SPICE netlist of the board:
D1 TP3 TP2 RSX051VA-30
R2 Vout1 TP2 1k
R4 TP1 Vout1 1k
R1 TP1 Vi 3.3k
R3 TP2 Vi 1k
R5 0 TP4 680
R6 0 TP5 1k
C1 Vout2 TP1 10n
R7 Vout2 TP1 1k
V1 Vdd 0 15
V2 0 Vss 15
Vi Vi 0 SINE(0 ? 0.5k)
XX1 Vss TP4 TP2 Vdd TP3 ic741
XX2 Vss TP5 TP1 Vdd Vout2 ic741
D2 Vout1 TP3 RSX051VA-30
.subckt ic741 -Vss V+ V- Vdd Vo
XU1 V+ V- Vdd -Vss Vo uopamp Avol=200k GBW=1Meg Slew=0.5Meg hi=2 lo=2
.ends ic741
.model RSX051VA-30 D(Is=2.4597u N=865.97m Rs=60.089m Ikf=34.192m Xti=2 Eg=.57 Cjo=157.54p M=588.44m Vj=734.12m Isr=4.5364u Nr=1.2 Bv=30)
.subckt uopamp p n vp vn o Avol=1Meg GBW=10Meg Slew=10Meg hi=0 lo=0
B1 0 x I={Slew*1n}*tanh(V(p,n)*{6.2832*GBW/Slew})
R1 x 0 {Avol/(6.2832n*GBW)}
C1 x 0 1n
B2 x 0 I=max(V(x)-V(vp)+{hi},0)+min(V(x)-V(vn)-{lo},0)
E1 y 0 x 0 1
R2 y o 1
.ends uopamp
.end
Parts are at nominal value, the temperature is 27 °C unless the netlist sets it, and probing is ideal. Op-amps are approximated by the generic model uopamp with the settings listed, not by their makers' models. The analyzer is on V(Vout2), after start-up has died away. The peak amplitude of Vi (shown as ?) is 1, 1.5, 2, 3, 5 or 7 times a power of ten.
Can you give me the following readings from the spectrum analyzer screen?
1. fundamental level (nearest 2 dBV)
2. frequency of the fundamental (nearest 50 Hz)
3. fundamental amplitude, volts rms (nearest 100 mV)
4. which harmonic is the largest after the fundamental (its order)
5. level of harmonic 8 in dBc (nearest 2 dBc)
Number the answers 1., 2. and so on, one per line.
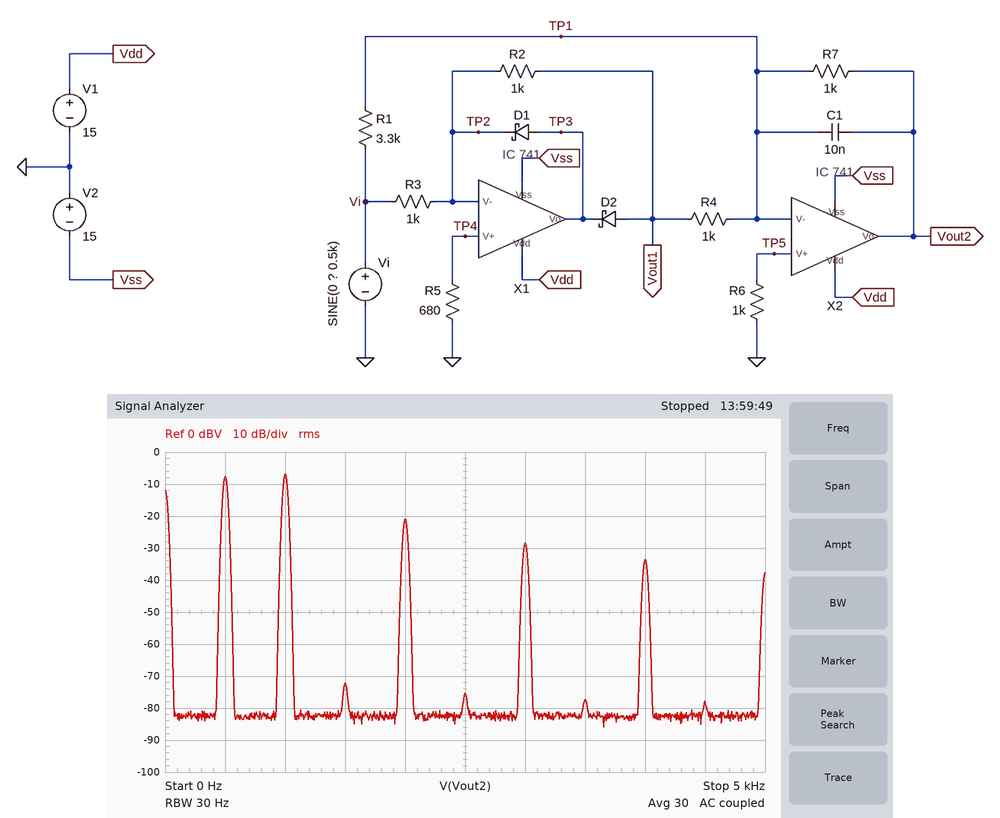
1. -8 dBV
2. 500 Hz
3. 400 mV
4. 2
5. -26 dBc
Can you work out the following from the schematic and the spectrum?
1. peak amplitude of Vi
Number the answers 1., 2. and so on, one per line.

1. 3 V
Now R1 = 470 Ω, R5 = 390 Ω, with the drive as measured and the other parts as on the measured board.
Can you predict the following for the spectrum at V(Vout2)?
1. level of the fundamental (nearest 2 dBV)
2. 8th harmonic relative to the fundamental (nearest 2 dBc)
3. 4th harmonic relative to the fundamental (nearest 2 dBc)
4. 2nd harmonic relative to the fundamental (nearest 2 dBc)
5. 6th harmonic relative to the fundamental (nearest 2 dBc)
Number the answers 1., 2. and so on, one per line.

1. 10 dBV
2. -44 dBc
3. -32 dBc
4. -18 dBc
5. -40 dBc
